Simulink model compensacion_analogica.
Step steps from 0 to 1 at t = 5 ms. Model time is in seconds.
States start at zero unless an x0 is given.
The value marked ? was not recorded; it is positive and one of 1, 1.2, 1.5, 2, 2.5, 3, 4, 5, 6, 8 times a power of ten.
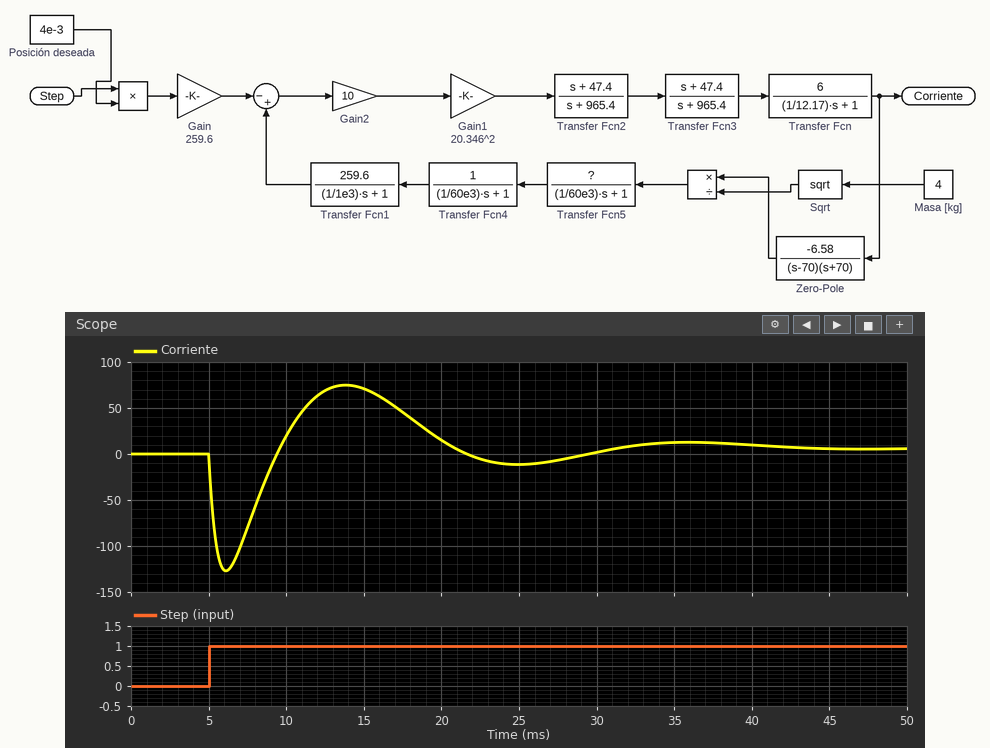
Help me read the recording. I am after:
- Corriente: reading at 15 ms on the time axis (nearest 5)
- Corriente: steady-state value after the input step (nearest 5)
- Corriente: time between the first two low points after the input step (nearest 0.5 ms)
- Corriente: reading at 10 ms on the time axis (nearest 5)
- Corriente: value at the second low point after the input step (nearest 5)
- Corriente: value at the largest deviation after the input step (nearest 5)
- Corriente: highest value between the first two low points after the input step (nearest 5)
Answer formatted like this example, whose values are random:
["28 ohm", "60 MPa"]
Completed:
["70", "5", "19.0 ms", "20", "-10", "-125", "75"]
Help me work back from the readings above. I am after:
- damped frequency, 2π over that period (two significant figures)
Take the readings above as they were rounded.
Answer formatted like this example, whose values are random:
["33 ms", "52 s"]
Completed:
["0.33 rad/ms"]
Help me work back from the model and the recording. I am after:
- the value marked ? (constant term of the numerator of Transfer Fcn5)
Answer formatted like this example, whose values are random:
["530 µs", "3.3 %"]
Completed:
["1"]
